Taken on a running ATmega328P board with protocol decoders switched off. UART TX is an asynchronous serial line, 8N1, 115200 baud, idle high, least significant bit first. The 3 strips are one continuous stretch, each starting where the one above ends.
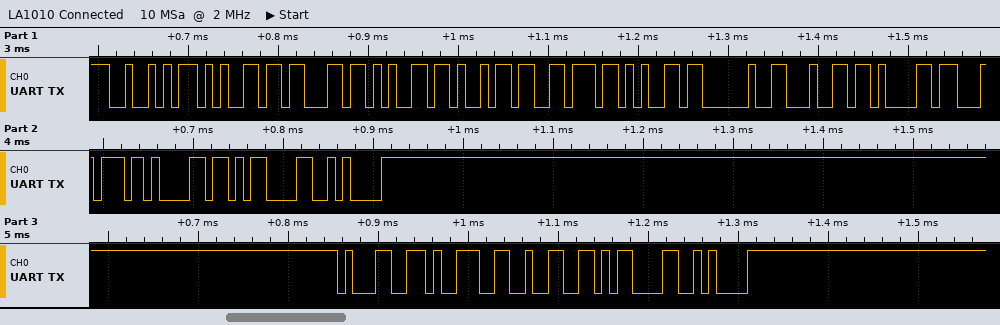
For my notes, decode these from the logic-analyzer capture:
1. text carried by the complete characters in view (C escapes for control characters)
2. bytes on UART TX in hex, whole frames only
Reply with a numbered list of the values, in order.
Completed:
1. "Receive data\r\n192\r\n"
2. 52 65 63 65 69 76 65 20 64 61 74 61 0D 0A 31 39 32 0D 0A
